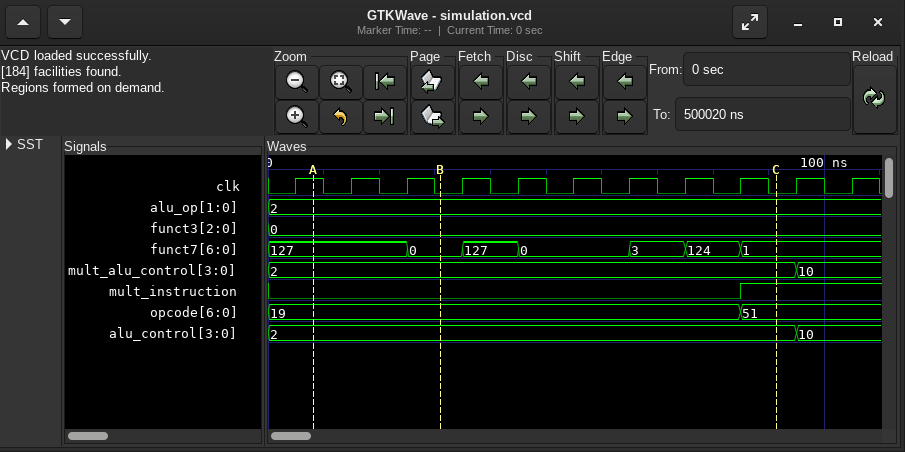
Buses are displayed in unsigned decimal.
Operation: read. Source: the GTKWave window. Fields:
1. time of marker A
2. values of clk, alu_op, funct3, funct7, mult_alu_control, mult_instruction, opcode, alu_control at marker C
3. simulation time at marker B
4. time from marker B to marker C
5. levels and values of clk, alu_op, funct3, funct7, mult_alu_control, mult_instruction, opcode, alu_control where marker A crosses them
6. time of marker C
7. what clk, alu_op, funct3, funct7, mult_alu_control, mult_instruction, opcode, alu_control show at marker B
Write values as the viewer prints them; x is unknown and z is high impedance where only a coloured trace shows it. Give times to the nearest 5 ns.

10 ns
clk=0, alu_op=2, funct3=0, funct7=1, mult_alu_control=2, mult_instruction=1, opcode=51, alu_control=2
30 ns
60 ns
clk=1, alu_op=2, funct3=0, funct7=127, mult_alu_control=2, mult_instruction=0, opcode=19, alu_control=2
90 ns
clk=0, alu_op=2, funct3=0, funct7=0, mult_alu_control=2, mult_instruction=0, opcode=19, alu_control=2
